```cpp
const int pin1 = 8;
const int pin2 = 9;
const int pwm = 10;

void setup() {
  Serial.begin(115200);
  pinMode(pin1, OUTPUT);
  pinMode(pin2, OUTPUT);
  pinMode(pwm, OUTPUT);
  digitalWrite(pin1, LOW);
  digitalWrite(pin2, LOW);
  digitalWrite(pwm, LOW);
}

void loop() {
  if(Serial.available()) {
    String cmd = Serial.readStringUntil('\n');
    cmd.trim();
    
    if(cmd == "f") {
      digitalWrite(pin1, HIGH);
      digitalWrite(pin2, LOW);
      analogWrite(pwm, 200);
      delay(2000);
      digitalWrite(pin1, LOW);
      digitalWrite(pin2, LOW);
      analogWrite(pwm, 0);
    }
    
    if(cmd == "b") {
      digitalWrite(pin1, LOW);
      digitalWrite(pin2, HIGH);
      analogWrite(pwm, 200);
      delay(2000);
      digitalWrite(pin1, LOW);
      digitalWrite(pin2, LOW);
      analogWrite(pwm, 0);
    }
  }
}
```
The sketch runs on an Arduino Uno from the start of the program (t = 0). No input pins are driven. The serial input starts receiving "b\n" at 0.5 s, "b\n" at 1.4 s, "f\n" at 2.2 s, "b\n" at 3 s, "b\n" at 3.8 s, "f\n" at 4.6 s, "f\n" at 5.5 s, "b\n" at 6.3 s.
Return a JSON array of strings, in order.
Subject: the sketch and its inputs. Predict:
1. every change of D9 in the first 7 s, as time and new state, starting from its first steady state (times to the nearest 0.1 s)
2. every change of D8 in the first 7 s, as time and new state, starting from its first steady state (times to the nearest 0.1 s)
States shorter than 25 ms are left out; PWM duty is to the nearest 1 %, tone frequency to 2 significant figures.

["0 s low; 0.5 s high; 4.5 s low; 6.5 s high", "0 s low; 4.5 s high; 6.5 s low"]
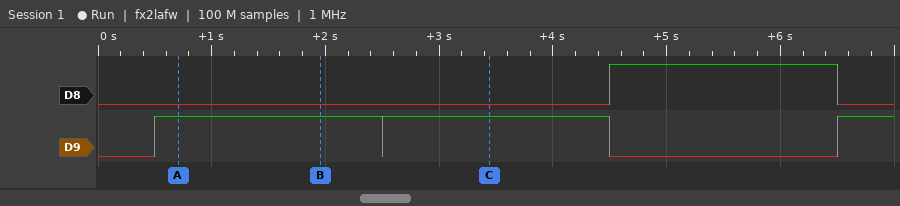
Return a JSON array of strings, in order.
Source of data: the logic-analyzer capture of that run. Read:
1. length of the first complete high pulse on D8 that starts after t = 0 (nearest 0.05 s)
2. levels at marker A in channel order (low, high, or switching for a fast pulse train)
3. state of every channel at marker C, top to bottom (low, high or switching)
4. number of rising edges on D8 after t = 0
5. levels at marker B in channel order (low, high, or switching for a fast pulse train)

["2.00 s", "D8 low, D9 high", "D8 low, D9 high", "1", "D8 low, D9 high"]
